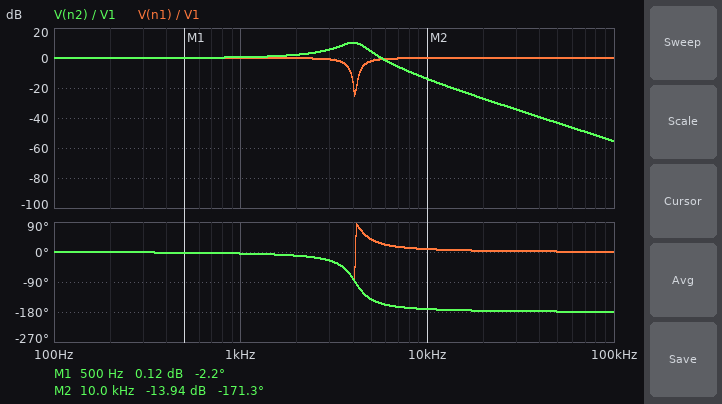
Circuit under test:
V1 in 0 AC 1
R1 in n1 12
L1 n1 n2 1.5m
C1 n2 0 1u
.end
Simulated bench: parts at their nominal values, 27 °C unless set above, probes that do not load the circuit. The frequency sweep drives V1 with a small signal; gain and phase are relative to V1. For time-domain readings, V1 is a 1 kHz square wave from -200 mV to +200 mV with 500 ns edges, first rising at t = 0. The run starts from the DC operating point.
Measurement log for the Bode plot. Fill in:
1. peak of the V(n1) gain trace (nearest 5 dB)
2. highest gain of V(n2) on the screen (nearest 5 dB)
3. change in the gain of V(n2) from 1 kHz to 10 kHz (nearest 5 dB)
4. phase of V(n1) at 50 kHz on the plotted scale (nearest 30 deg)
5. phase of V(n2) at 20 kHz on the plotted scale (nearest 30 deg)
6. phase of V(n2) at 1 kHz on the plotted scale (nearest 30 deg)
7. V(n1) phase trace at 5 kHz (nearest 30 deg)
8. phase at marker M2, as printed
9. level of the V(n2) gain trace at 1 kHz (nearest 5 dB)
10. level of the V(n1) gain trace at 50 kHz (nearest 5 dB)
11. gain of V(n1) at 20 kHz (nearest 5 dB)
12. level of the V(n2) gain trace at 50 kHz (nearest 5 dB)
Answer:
0 dB
10 dB
-15 dB
0 deg
-180 deg
0 deg
30 deg
-171.3 deg
0 dB
0 dB
0 dB
-45 dB
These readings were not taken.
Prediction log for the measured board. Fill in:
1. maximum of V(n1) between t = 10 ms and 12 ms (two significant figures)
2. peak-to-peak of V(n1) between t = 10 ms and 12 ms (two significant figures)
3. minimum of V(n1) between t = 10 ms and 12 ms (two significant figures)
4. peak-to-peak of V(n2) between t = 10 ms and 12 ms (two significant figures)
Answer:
250 mV
510 mV
-250 mV
830 mV
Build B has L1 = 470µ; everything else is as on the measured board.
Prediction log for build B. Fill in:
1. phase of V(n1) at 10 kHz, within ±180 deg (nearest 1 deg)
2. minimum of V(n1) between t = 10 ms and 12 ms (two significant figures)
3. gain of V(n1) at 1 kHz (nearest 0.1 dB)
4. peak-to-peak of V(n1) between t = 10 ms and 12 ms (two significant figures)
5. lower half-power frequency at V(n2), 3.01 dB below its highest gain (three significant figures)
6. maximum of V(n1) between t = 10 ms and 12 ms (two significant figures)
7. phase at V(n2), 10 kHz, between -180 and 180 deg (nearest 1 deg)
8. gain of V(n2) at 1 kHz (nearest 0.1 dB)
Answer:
41 deg
-260 mV
0 dB
520 mV
4.12 kHz
260 mV
-139 deg
0.1 dB
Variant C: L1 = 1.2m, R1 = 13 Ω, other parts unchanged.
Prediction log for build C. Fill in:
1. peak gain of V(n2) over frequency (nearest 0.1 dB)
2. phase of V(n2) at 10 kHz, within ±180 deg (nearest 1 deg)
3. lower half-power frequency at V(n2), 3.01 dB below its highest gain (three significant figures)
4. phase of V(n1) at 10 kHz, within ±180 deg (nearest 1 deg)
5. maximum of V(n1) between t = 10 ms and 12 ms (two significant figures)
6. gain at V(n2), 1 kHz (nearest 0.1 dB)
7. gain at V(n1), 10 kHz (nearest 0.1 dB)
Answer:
8.7 dB
-168 deg
3.44 kHz
12 deg
260 mV
0.4 dB
-0.2 dB
